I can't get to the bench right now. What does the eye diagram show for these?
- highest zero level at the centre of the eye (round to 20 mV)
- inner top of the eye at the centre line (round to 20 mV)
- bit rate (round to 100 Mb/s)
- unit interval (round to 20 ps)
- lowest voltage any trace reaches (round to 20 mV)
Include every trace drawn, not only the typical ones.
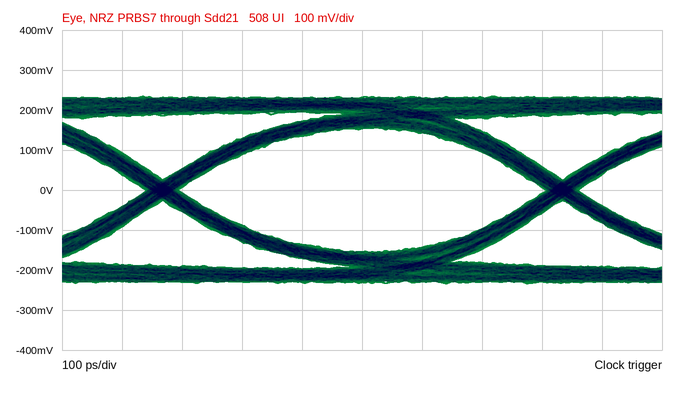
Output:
-160 mV
160 mV
1.5 Gb/s
660 ps
-240 mV
